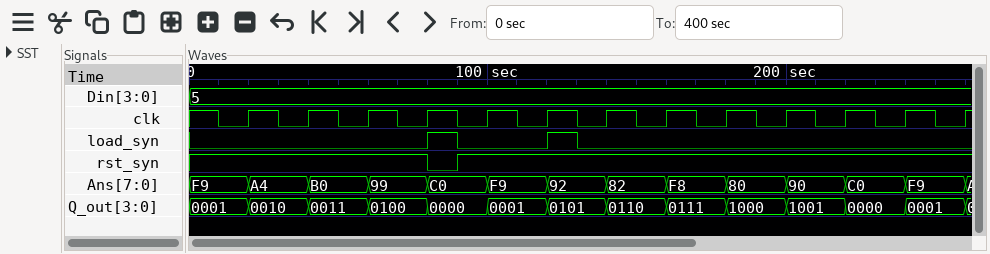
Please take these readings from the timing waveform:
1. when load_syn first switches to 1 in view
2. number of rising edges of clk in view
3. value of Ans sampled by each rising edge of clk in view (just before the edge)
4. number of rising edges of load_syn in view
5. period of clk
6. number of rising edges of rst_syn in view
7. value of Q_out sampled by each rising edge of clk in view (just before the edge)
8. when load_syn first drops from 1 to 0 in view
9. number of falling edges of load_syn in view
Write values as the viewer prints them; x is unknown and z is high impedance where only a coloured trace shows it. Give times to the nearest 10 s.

80 s
13
F9, A4, B0, 99, C0, F9, 92, 82, F8, 80, 90, C0, F9
2
20 s
1
0001, 0010, 0011, 0100, 0000, 0001, 0101, 0110, 0111, 1000, 1001, 0000, 0001
90 s
2
